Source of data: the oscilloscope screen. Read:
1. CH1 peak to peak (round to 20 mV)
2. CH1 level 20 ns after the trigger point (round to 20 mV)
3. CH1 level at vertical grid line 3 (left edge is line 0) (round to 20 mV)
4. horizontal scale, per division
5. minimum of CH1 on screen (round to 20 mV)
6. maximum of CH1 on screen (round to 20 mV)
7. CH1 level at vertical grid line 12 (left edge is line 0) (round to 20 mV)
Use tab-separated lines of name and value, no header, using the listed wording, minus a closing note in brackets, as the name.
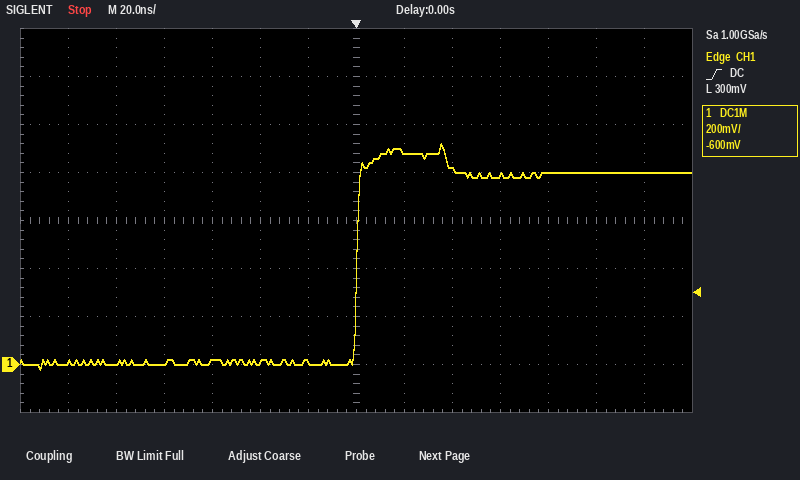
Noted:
CH1 peak to peak	940 mV
CH1 level 20 ns after the trigger point	880 mV
CH1 level at vertical grid line 3 (left edge is line 0)	0 mV
horizontal scale, per division	20 ns
minimum of CH1 on screen	-20 mV
maximum of CH1 on screen	920 mV
CH1 level at vertical grid line 12 (left edge is line 0)	800 mV
